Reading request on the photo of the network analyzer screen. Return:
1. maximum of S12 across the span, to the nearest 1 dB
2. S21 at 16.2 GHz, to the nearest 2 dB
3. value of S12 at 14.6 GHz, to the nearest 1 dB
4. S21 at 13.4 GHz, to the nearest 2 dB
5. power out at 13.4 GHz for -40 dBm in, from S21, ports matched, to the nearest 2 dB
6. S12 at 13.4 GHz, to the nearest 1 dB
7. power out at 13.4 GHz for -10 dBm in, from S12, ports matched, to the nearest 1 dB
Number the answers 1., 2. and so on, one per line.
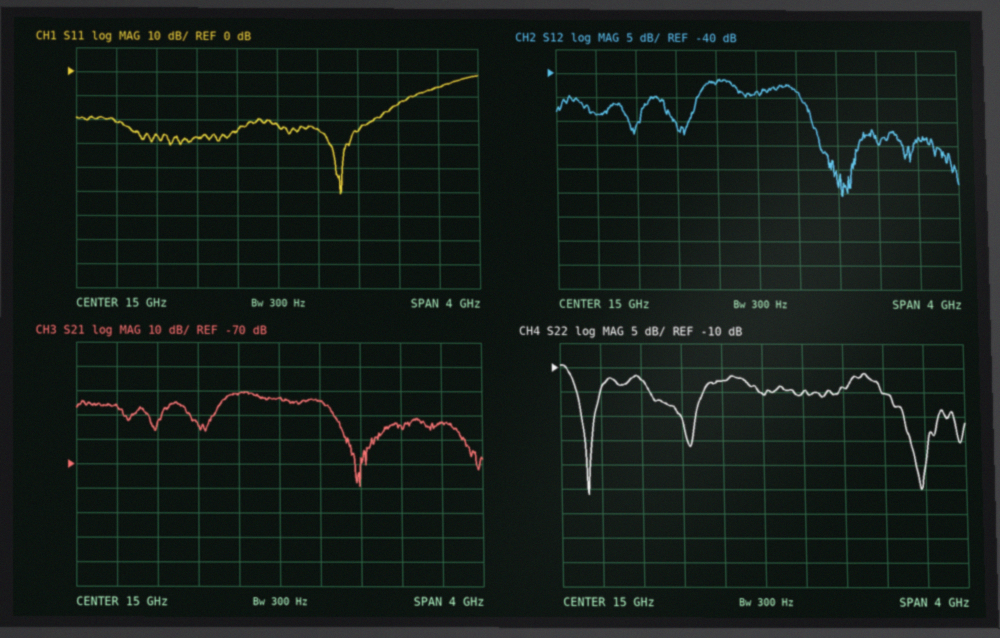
1. -41 dB
2. -54 dB
3. -42 dB
4. -46 dB
5. -86 dBm
6. -49 dB
7. -59 dBm
